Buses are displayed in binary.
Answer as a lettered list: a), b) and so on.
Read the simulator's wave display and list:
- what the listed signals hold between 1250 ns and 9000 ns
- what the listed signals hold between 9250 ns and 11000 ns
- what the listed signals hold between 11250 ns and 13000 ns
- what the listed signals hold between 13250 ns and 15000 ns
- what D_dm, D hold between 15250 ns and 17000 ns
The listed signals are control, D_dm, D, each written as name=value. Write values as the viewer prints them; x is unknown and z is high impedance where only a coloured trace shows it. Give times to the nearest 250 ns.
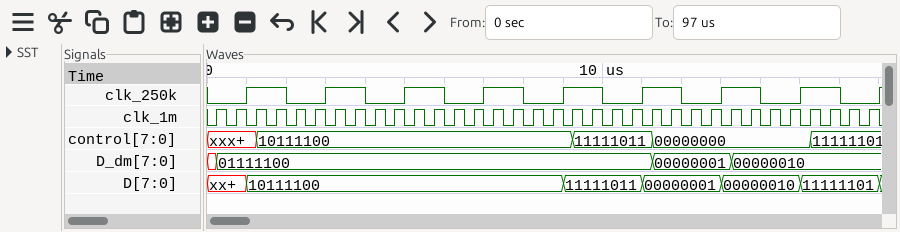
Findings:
a) control=10111100, D_dm=01111100, D=10111100
b) control=11111011, D_dm=01111100, D=11111011
c) control=00000000, D_dm=00000001, D=00000001
d) control=00000000, D_dm=00000010, D=00000010
e) D_dm=00000010, D=11111101
